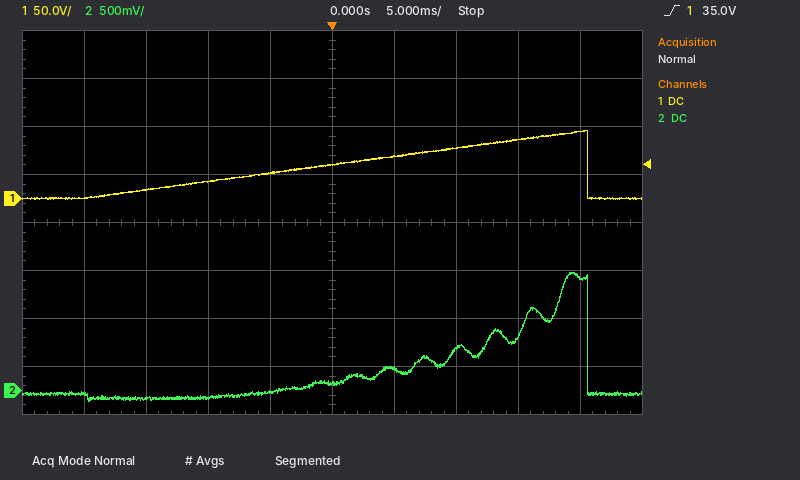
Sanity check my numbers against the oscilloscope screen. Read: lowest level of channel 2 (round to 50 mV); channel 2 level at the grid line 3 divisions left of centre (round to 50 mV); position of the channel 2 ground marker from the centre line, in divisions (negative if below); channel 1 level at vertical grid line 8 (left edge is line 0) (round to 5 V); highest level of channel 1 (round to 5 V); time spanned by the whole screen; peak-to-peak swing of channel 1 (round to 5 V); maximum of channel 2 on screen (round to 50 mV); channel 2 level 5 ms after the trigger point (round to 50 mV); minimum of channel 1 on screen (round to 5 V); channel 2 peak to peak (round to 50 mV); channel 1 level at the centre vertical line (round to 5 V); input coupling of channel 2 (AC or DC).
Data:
-100 mV
-100 mV
-3.5 div
60 V
70 V
50 ms
70 V
1.25 V
200 mV
0 V
1.35 V
35 V
DC
